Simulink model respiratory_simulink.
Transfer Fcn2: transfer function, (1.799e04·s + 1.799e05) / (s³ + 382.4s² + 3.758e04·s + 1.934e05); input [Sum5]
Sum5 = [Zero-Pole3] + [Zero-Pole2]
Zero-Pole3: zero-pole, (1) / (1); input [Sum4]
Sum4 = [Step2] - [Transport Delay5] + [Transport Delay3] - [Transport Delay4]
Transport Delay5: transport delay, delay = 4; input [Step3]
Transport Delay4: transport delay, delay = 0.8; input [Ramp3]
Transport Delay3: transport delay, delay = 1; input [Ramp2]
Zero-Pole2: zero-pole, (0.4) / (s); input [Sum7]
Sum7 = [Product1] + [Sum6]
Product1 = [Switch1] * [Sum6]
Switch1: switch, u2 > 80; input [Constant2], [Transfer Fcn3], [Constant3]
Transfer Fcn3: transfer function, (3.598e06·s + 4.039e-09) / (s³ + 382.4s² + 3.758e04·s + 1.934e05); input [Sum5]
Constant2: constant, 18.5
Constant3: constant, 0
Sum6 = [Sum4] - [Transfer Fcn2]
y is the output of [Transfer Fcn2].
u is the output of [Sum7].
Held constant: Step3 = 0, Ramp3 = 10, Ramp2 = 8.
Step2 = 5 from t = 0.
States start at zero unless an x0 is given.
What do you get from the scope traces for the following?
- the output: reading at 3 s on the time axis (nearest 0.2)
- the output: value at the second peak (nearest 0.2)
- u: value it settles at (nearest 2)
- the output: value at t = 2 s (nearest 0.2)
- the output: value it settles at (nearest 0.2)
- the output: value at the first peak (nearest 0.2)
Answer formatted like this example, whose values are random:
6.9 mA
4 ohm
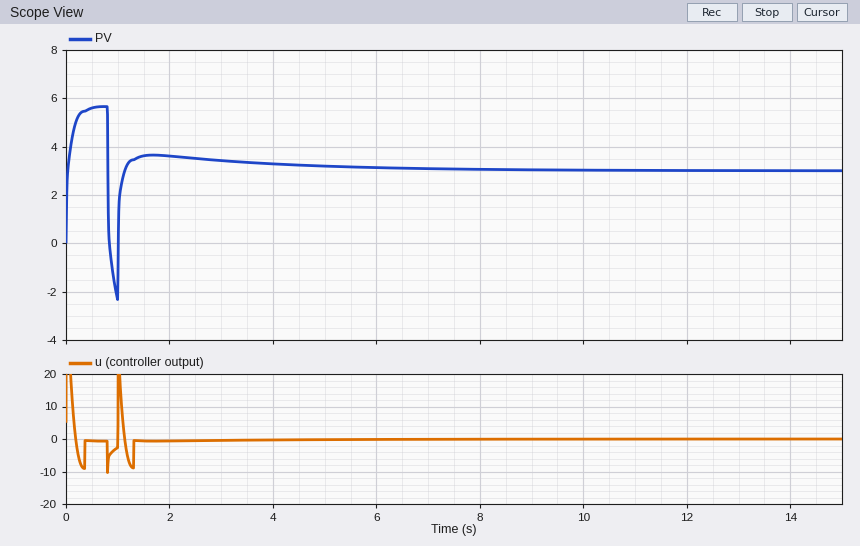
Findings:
3.4
3.6
0
3.6
3.0
5.6
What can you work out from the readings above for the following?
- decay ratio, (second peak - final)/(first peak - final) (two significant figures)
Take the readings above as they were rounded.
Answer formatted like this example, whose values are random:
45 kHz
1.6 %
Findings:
0.23
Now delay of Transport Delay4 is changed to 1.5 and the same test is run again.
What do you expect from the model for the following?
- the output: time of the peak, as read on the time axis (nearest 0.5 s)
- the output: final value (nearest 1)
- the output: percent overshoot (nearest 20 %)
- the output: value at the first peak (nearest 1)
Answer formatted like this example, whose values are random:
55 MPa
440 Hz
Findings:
1.5 s
3
360 %
14
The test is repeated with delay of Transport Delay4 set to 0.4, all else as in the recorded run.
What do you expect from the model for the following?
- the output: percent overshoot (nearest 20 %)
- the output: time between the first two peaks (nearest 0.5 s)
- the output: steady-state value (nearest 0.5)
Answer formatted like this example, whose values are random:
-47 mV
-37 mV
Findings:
80 %
1.5 s
3.0
